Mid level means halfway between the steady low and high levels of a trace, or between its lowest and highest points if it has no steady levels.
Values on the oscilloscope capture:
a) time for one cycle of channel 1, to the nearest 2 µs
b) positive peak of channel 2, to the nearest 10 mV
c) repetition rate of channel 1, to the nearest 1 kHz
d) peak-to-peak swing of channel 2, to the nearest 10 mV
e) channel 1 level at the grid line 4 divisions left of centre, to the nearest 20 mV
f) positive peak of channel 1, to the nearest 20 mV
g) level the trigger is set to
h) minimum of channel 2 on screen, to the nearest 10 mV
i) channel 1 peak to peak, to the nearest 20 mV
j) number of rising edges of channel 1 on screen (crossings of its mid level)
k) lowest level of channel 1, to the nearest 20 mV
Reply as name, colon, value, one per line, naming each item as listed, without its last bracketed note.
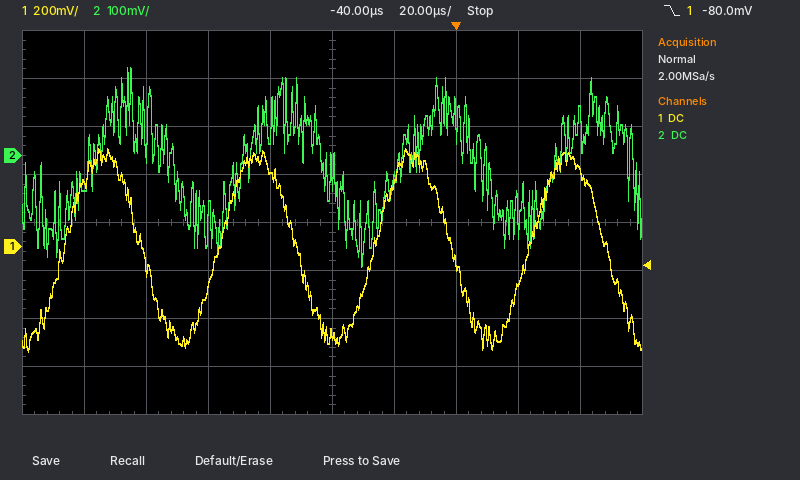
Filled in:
time for one cycle of channel 1, to the nearest 2 µs: 50 µs
positive peak of channel 2, to the nearest 10 mV: 180 mV
repetition rate of channel 1, to the nearest 1 kHz: 20 kHz
peak-to-peak swing of channel 2, to the nearest 10 mV: 410 mV
channel 1 level at the grid line 4 divisions left of centre, to the nearest 20 mV: 260 mV
positive peak of channel 1, to the nearest 20 mV: 400 mV
level the trigger is set to: -80.0 mV
minimum of channel 2 on screen, to the nearest 10 mV: -230 mV
channel 1 peak to peak, to the nearest 20 mV: 840 mV
number of rising edges of channel 1 on screen: 4
lowest level of channel 1, to the nearest 20 mV: -440 mV
